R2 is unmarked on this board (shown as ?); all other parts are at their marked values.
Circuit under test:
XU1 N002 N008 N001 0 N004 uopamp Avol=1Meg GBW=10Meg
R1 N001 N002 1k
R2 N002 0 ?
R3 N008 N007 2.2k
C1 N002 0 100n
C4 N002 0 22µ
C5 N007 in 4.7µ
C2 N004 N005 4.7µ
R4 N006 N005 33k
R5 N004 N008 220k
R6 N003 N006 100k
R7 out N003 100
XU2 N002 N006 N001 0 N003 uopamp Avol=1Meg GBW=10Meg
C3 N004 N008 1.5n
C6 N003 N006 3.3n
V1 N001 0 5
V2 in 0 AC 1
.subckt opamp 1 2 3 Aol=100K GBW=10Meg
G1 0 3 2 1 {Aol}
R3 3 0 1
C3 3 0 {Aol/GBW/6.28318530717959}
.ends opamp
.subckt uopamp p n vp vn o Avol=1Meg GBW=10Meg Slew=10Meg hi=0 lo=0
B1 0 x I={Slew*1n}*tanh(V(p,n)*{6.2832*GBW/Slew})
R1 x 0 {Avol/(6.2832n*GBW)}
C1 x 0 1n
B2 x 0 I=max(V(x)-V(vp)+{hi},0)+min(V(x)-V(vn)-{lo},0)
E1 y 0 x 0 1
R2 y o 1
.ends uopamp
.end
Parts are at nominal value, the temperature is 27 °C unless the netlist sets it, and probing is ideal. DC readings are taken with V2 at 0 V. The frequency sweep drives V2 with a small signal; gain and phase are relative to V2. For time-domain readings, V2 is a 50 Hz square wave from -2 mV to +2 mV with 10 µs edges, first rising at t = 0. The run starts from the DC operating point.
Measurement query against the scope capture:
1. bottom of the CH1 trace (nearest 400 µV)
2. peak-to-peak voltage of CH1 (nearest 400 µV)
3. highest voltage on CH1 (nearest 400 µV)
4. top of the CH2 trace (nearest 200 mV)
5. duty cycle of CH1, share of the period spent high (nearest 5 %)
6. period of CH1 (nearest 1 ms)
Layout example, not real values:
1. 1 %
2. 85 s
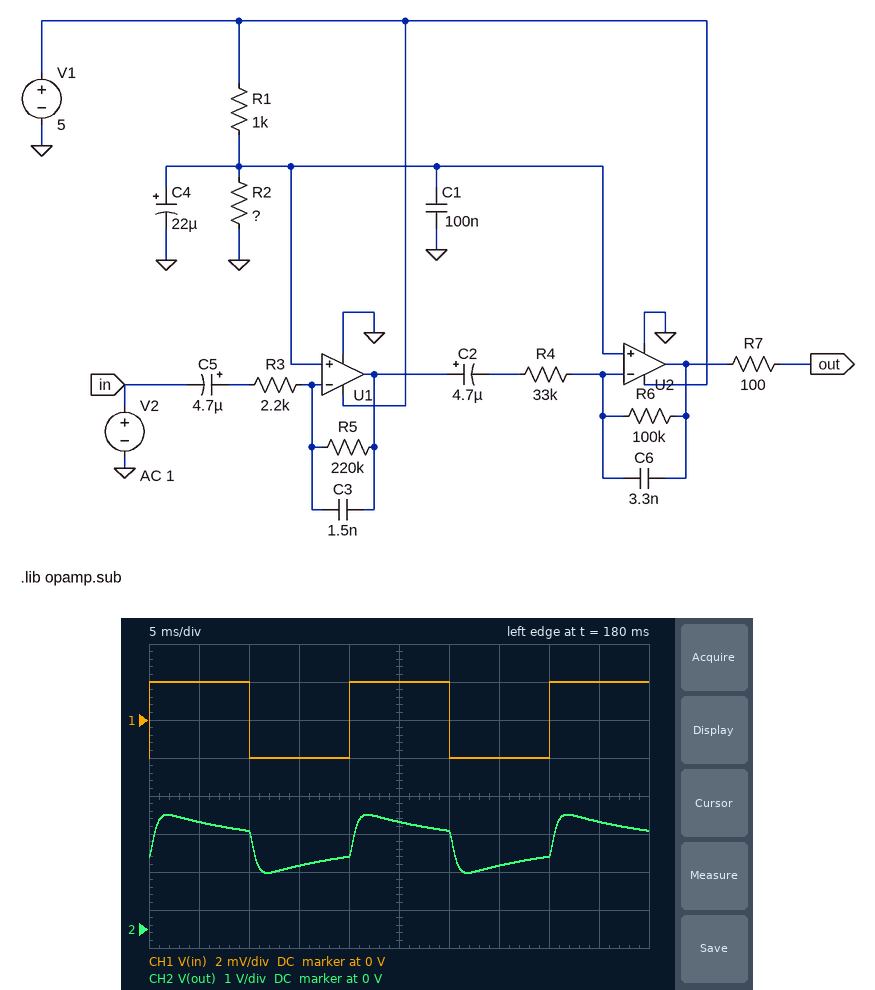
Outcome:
1. -2.0 mV
2. 4.0 mV
3. 2.0 mV
4. 3.0 V
5. 50 %
6. 20 ms
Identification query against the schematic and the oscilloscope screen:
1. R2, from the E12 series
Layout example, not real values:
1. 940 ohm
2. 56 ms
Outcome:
1. 820 Ω
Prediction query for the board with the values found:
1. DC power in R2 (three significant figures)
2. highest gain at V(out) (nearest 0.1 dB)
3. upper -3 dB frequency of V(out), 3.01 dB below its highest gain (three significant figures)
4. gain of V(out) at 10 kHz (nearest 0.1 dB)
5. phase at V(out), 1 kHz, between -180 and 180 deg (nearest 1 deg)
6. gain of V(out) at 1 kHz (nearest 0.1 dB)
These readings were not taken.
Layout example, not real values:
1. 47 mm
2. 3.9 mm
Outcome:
1. 6.19 mW
2. 49.2 dB
3. 332 Hz
4. -3.1 dB
5. -128 deg
6. 35.1 dB
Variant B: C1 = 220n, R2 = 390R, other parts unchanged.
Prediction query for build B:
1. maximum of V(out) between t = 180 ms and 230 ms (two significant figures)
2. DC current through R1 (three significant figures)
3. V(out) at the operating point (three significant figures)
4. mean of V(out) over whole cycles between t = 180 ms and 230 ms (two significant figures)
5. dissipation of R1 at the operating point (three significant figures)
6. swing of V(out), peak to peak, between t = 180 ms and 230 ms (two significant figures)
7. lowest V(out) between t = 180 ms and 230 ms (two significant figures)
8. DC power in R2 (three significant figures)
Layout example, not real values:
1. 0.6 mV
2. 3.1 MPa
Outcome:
1. 2.2 V
2. 3.60 mA
3. 1.40 V
4. 1.4 V
5. 12.9 mW
6. 1.5 V
7. 630 mV
8. 5.05 mW
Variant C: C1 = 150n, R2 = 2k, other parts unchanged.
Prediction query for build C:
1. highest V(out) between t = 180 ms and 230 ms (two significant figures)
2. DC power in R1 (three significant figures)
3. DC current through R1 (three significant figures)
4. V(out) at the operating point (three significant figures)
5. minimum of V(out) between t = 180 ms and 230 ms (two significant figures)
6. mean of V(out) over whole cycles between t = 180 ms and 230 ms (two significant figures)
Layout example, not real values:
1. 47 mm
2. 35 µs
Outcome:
1. 4.1 V
2. 2.78 mW
3. 1.67 mA
4. 3.33 V
5. 2.6 V
6. 3.3 V
